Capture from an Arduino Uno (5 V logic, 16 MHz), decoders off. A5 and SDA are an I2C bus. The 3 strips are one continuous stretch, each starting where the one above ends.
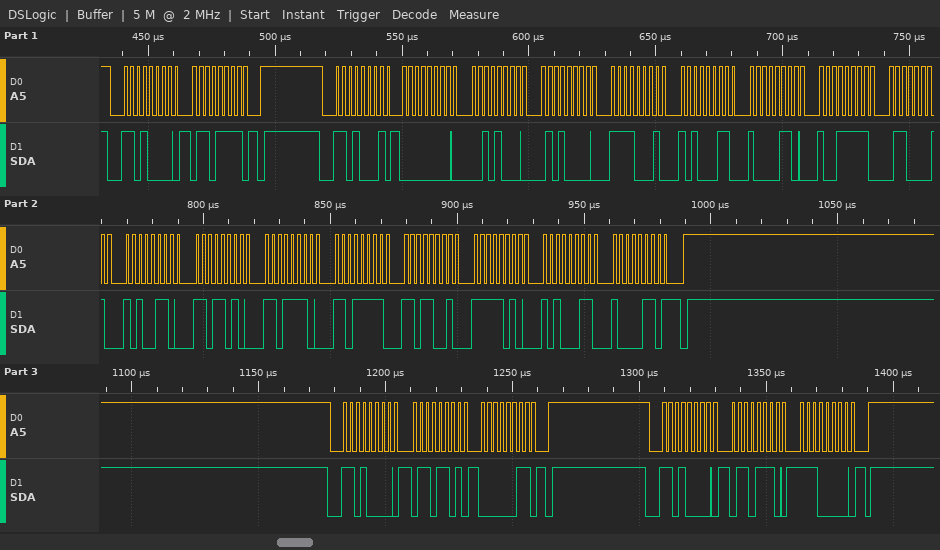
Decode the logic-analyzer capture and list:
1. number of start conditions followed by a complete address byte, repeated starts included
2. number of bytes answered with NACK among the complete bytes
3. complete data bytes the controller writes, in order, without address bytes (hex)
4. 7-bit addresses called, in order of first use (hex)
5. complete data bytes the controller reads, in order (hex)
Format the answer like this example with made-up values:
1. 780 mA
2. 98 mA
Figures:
1. 4
2. 1
3. 6F 6D 03 6E E0
4. 0x68
5. 00 28 50 F1 A3 86 9F 61 A6 DA DE DF D9 FA A3 86
